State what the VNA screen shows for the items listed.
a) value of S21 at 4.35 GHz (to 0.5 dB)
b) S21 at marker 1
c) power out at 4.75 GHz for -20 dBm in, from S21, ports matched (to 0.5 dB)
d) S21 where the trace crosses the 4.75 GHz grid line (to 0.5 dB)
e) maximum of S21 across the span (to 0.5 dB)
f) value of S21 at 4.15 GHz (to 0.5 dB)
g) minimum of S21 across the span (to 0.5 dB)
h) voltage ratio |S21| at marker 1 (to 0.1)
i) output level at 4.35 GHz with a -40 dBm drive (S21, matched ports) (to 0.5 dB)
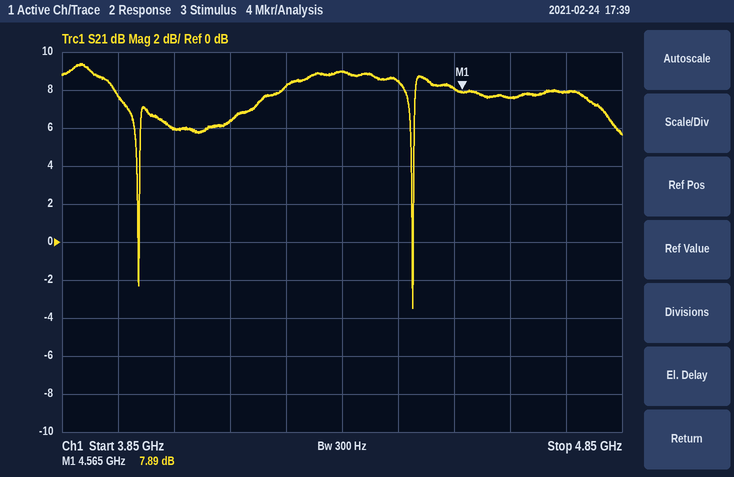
9.0 dB
7.89 dB
-12.0 dBm
8.0 dB
9.5 dB
6.5 dB
-3.5 dB
2.5
-31.0 dBm
